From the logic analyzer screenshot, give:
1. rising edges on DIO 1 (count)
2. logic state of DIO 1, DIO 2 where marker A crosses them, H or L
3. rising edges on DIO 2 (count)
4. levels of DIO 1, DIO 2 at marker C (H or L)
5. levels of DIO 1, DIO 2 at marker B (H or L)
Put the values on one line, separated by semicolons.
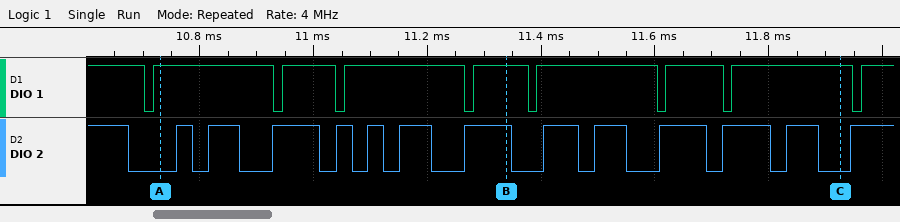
8; DIO 1=H, DIO 2=L; 13; DIO 1=H, DIO 2=L; DIO 1=H, DIO 2=H
